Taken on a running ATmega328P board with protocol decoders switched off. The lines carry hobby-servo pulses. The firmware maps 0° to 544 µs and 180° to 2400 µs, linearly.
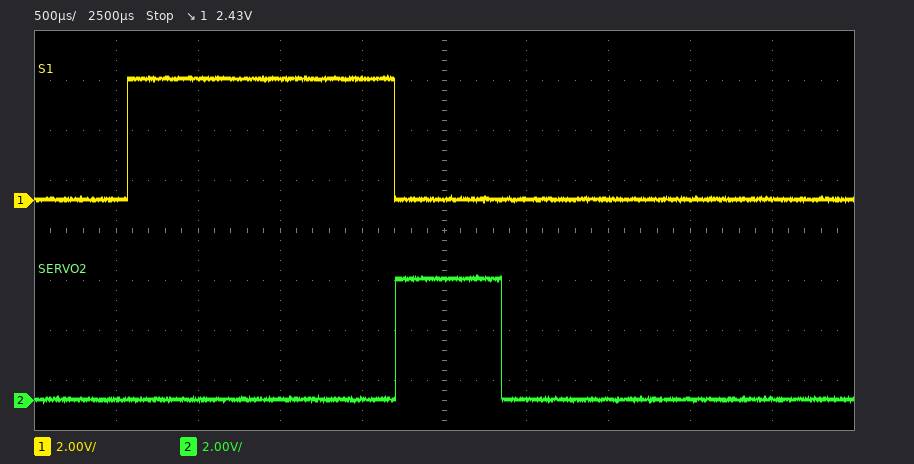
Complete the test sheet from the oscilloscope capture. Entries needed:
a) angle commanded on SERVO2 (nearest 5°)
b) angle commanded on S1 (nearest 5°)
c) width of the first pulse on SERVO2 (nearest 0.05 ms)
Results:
10°
105°
0.65 ms
